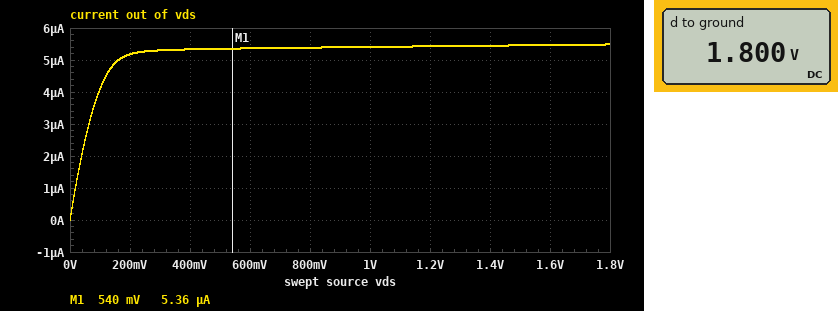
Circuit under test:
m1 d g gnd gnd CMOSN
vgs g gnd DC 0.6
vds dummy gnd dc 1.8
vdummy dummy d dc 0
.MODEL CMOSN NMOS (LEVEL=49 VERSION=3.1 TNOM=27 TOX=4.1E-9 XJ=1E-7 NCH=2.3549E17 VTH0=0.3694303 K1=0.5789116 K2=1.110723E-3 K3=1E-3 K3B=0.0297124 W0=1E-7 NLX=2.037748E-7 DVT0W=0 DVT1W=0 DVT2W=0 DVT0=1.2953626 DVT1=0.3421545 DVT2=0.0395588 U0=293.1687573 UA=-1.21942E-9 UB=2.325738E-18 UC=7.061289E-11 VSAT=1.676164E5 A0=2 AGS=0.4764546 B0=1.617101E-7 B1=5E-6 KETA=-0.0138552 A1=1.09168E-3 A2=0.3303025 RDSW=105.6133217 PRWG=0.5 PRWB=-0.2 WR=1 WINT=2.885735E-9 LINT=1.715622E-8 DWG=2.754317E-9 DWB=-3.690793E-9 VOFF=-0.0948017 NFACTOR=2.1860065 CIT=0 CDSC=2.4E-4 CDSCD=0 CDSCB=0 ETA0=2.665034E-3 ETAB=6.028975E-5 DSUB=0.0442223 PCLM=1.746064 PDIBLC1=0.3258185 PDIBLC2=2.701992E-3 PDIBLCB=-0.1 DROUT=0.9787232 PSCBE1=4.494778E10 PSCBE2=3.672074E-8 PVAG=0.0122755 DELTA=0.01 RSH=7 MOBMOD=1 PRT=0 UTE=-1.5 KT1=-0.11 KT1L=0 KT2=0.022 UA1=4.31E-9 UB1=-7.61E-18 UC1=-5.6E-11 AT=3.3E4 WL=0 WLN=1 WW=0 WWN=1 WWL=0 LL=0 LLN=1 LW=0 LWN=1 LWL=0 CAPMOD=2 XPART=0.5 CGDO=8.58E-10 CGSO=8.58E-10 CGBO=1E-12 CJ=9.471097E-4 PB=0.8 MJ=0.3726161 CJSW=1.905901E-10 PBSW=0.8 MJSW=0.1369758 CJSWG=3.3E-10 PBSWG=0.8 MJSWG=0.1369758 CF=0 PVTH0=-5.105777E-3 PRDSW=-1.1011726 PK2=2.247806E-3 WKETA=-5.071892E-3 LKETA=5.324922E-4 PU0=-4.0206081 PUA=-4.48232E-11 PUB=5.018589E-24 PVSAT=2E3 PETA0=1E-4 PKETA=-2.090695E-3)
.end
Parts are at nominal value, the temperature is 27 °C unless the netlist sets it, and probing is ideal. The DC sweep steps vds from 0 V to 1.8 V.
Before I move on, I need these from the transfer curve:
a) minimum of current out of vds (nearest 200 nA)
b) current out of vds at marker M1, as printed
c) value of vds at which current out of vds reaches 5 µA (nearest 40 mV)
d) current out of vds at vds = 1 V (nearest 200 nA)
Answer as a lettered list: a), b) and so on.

a) 0 A
b) 5.36 µA
c) 160 mV
d) 5.4 µA
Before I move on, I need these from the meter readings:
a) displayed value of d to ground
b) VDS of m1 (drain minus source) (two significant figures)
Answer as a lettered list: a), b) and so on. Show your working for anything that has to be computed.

a) 1.800 V
b) 1.8 V = 1.8 V
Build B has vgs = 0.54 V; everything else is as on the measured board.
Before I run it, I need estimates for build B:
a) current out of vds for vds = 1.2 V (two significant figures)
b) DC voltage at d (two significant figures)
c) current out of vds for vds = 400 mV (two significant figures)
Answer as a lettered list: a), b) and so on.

a) 2.9 µA
b) 1.8 V
c) 2.8 µA
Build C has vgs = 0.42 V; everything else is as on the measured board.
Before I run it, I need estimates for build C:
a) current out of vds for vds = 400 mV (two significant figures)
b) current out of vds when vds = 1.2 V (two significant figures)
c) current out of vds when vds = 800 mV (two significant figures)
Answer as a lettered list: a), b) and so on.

a) 390 nA
b) 410 nA
c) 400 nA
